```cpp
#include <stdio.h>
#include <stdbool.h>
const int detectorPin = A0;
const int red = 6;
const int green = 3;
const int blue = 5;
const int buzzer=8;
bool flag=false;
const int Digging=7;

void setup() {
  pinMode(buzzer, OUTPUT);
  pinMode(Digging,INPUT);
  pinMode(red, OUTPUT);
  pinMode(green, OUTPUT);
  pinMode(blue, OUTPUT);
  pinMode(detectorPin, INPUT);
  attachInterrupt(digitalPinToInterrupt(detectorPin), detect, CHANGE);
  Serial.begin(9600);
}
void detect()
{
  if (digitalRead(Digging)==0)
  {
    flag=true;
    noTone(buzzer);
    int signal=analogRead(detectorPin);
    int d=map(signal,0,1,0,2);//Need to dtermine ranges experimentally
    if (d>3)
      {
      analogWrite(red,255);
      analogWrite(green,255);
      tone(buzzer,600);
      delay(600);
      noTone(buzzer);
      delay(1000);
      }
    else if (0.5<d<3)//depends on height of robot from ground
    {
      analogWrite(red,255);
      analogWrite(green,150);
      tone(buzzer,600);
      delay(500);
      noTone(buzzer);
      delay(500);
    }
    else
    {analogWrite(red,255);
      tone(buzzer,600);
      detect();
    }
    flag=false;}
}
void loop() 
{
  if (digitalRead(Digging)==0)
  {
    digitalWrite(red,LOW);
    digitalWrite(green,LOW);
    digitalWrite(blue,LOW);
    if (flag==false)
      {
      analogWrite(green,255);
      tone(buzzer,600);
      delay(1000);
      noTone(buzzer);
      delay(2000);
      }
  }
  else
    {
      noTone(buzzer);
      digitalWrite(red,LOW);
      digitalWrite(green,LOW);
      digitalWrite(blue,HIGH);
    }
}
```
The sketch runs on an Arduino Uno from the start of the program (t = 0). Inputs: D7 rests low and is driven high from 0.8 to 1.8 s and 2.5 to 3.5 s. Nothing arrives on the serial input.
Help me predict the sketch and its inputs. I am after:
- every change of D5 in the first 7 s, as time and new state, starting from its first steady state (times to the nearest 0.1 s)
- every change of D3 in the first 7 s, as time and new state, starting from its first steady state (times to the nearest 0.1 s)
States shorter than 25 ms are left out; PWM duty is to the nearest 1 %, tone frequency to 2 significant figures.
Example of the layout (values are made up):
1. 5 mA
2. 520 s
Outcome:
1. 0 s low; 3 s high; 3.5 s low
2. 0 s high; 3 s low; 3.5 s high
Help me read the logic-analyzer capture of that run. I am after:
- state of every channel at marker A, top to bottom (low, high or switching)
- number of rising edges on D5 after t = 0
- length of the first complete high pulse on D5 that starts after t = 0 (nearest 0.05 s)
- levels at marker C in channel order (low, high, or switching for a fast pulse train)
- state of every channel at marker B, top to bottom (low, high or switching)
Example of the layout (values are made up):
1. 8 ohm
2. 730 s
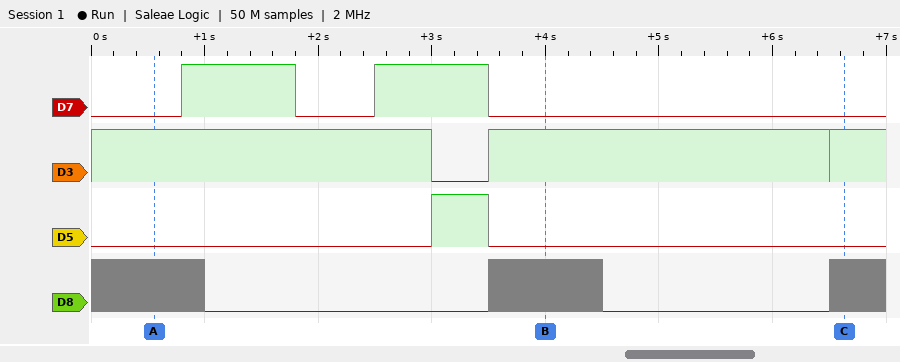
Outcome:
1. D7 low, D3 high, D5 low, D8 switching
2. 1
3. 0.50 s
4. D7 low, D3 high, D5 low, D8 switching
5. D7 low, D3 high, D5 low, D8 switching
